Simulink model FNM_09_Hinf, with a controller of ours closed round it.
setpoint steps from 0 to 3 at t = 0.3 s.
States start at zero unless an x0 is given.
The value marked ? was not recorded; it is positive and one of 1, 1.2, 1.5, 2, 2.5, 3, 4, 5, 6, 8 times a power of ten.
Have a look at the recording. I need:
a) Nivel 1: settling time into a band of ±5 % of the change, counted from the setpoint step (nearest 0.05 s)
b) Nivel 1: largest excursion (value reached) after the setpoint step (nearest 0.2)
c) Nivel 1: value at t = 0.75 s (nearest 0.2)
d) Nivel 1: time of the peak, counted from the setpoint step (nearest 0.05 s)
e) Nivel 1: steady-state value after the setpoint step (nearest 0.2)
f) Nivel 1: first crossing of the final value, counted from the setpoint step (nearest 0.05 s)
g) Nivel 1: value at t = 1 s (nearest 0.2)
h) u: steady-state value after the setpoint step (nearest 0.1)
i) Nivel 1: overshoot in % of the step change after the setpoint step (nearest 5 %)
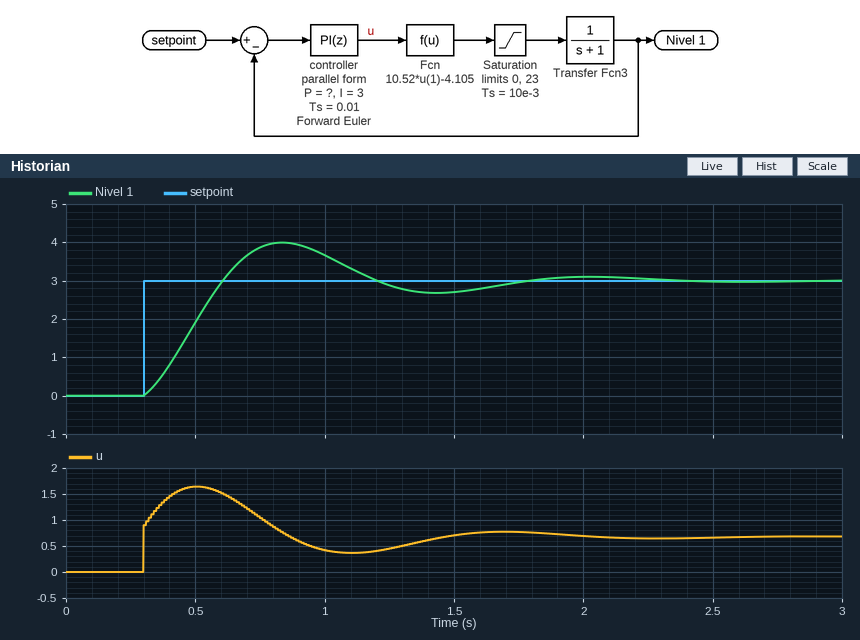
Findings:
1.35 s
4.0
3.8
0.55 s
3.0
0.30 s
3.6
0.7
35 %
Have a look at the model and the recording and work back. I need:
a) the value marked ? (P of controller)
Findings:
0.3
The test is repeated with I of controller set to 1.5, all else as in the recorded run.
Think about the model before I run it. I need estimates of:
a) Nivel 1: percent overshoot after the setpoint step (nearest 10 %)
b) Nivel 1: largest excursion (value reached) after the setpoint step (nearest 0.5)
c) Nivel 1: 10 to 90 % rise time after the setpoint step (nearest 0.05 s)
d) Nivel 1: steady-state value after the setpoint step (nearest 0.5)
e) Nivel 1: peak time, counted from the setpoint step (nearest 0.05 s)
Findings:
20 %
3.5
0.35 s
3.0
0.80 s
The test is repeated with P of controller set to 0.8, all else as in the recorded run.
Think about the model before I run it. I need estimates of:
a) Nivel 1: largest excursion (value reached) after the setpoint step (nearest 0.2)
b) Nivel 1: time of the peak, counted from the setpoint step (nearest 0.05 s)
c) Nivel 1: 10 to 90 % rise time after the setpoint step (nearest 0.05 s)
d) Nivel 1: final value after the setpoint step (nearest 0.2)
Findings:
3.2
0.45 s
0.20 s
3.0
